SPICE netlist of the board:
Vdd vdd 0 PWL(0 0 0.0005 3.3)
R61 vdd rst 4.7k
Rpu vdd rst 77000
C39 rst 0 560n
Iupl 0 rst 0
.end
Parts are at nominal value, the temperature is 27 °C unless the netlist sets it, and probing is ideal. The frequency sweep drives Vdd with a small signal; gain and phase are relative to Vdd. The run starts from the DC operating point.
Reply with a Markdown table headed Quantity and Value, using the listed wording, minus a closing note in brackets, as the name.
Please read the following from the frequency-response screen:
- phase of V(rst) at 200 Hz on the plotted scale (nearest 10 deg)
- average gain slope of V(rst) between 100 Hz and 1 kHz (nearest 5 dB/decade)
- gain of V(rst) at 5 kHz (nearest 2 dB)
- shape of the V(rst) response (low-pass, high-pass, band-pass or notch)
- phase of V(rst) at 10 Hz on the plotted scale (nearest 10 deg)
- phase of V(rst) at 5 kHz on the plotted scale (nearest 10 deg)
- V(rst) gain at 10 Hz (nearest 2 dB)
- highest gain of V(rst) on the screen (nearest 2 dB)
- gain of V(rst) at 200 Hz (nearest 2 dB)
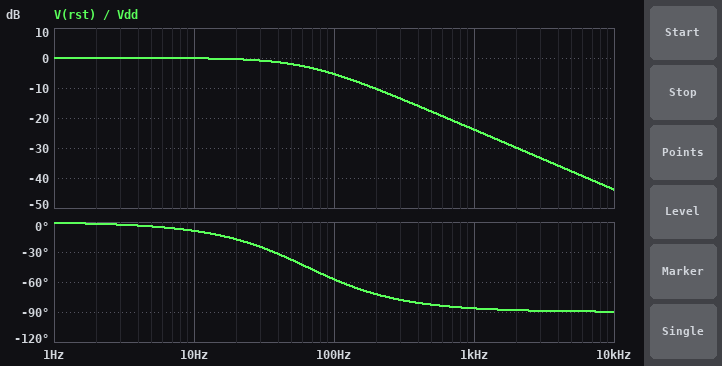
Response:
| Quantity | Value |
|---|---|
| phase of V(rst) at 200 Hz on the plotted scale | -70 deg |
| average gain slope of V(rst) between 100 Hz and 1 kHz | -20 dB/decade |
| gain of V(rst) at 5 kHz | -38 dB |
| shape of the V(rst) response | low-pass |
| phase of V(rst) at 10 Hz on the plotted scale | -10 deg |
| phase of V(rst) at 5 kHz on the plotted scale | -90 deg |
| V(rst) gain at 10 Hz | 0 dB |
| highest gain of V(rst) on the screen | 0 dB |
| gain of V(rst) at 200 Hz | -10 dB |
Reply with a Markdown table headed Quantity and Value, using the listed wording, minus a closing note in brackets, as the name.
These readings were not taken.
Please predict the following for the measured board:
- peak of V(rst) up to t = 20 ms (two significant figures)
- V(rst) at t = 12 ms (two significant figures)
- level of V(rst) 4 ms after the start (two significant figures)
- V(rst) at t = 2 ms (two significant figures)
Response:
| Quantity | Value |
|---|---|
| peak of V(rst) up to t = 20 ms | 3.3 V |
| V(rst) at t = 12 ms | 3.3 V |
| level of V(rst) 4 ms after the start | 2.6 V |
| V(rst) at t = 2 ms | 1.7 V |
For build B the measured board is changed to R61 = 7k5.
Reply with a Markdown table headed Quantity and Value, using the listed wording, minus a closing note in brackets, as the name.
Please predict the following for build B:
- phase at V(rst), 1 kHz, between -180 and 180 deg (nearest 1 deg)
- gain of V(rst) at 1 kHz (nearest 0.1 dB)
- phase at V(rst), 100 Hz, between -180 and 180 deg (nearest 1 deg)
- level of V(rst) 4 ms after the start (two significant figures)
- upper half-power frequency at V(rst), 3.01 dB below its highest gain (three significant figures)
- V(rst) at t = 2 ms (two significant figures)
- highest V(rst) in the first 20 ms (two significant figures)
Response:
| Quantity | Value |
|---|---|
| phase at V(rst), 1 kHz, between -180 and 180 deg | -88 deg |
| gain of V(rst) at 1 kHz | -27.6 dB |
| phase at V(rst), 100 Hz, between -180 and 180 deg | -67 deg |
| level of V(rst) 4 ms after the start | 2.1 V |
| upper half-power frequency at V(rst), 3.01 dB below its highest gain | 41.6 Hz |
| V(rst) at t = 2 ms | 1.2 V |
| highest V(rst) in the first 20 ms | 3.3 V |
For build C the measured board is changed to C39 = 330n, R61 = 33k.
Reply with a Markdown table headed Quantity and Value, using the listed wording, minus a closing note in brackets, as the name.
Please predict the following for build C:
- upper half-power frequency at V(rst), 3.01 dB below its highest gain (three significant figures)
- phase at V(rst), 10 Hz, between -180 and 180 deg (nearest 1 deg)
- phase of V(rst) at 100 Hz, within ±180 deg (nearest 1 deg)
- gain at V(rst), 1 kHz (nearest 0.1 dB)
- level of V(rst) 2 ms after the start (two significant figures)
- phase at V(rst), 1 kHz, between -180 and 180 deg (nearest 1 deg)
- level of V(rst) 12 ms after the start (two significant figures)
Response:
| Quantity | Value |
|---|---|
| upper half-power frequency at V(rst), 3.01 dB below its highest gain | 20.9 Hz |
| phase at V(rst), 10 Hz, between -180 and 180 deg | -26 deg |
| phase of V(rst) at 100 Hz, within ±180 deg | -78 deg |
| gain at V(rst), 1 kHz | -33.6 dB |
| level of V(rst) 2 ms after the start | 680 mV |
| phase at V(rst), 1 kHz, between -180 and 180 deg | -89 deg |
| level of V(rst) 12 ms after the start | 2.6 V |
